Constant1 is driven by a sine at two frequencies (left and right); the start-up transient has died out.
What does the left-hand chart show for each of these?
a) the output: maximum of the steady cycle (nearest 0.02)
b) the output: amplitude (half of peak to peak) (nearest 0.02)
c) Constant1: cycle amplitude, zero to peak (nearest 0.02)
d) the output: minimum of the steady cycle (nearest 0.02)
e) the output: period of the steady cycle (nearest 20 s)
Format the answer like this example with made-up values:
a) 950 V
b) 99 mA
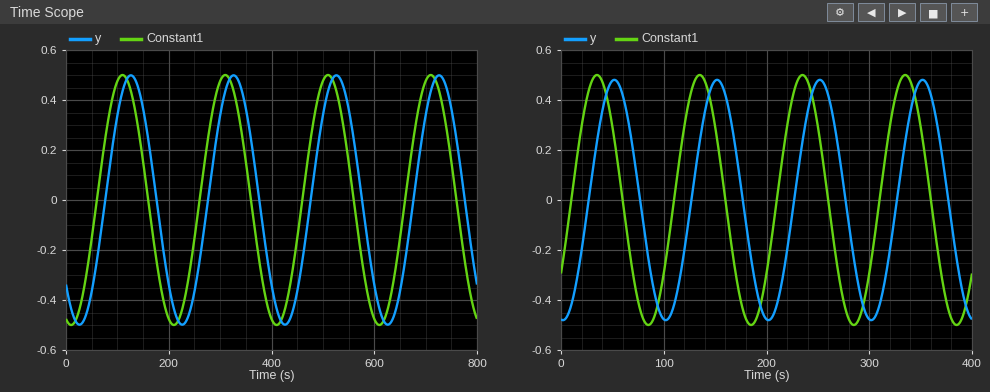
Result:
a) 0.50
b) 0.50
c) 0.50
d) -0.50
e) 200 s
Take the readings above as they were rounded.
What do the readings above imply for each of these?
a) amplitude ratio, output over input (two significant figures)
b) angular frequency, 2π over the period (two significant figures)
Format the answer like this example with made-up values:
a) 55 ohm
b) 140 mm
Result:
a) 1.0
b) 0.031 rad/s
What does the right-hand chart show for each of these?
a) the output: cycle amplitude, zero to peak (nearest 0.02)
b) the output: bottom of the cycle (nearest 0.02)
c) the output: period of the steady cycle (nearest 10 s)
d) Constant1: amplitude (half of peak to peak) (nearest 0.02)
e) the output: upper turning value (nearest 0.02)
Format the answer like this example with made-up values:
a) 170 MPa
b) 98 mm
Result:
a) 0.48
b) -0.48
c) 100 s
d) 0.50
e) 0.48
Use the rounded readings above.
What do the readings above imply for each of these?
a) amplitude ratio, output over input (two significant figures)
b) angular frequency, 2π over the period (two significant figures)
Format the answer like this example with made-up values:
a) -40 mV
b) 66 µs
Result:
a) 0.96
b) 0.063 rad/s
